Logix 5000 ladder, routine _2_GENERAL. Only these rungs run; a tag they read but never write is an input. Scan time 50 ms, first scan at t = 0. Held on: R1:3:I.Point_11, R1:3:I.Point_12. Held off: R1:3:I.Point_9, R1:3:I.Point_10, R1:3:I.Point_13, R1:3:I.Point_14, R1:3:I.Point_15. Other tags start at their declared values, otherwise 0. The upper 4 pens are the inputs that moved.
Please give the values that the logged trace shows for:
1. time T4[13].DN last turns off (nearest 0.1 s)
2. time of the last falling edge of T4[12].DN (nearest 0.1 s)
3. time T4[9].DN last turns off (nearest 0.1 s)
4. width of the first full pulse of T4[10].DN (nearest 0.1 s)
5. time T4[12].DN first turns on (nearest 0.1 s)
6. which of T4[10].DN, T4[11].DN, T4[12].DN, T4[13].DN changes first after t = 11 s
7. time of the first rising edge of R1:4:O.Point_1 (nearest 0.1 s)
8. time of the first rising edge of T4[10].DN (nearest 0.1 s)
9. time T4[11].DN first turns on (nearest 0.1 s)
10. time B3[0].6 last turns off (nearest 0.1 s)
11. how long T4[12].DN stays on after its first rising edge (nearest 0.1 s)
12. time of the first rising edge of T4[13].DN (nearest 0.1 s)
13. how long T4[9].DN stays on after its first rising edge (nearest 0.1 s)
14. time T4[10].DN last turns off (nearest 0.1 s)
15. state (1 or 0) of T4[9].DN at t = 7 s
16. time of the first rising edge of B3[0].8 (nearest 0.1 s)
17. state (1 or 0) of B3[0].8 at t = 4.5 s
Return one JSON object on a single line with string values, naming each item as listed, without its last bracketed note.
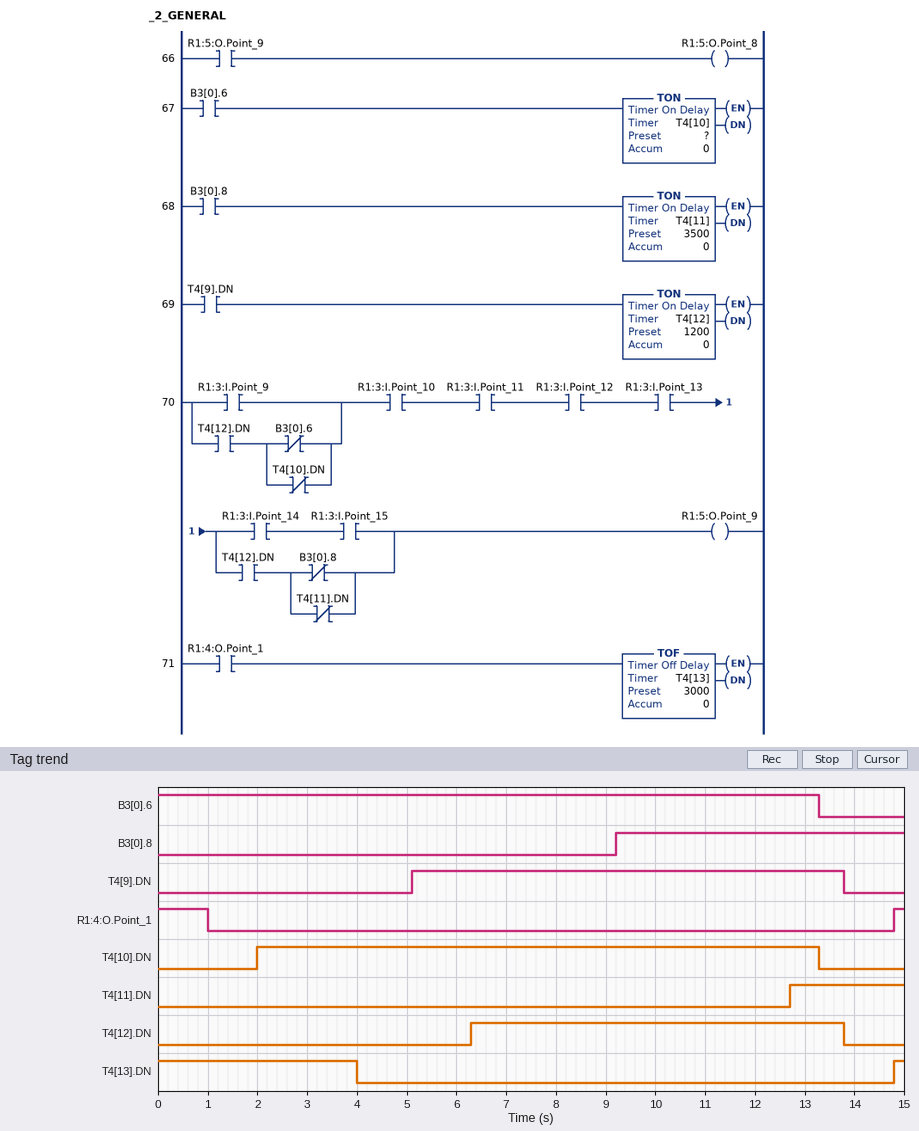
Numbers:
{"time T4[13].DN last turns off": "4.0 s", "time of the last falling edge of T4[12].DN": "13.8 s", "time T4[9].DN last turns off": "13.8 s", "width of the first full pulse of T4[10].DN": "11.3 s", "time T4[12].DN first turns on": "6.3 s", "which of T4[10].DN, T4[11].DN, T4[12].DN, T4[13].DN changes first after t = 11 s": "T4[11].DN", "time of the first rising edge of R1:4:O.Point_1": "14.8 s", "time of the first rising edge of T4[10].DN": "2.0 s", "time T4[11].DN first turns on": "12.7 s", "time B3[0].6 last turns off": "13.3 s", "how long T4[12].DN stays on after its first rising edge": "7.5 s", "time of the first rising edge of T4[13].DN": "14.8 s", "how long T4[9].DN stays on after its first rising edge": "8.7 s", "time T4[10].DN last turns off": "13.3 s", "state (1 or 0) of T4[9].DN at t = 7 s": "1", "time of the first rising edge of B3[0].8": "9.2 s", "state (1 or 0) of B3[0].8 at t = 4.5 s": "0"}
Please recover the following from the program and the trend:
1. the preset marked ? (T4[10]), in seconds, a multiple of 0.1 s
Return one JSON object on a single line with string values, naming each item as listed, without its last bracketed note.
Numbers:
{"the preset marked ? (T4[10]), in seconds, a multiple of 0.1 s": "2.0 s"}
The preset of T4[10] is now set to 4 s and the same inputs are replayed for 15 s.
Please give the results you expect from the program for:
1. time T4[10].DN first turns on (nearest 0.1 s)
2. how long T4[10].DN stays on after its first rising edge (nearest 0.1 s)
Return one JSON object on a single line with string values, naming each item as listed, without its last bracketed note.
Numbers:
{"time T4[10].DN first turns on": "4.0 s", "how long T4[10].DN stays on after its first rising edge": "9.3 s"}
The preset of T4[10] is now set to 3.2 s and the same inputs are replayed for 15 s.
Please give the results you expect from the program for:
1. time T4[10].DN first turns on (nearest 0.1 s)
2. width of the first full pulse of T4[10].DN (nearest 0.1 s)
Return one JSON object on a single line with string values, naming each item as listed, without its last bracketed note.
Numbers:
{"time T4[10].DN first turns on": "3.2 s", "width of the first full pulse of T4[10].DN": "10.1 s"}
